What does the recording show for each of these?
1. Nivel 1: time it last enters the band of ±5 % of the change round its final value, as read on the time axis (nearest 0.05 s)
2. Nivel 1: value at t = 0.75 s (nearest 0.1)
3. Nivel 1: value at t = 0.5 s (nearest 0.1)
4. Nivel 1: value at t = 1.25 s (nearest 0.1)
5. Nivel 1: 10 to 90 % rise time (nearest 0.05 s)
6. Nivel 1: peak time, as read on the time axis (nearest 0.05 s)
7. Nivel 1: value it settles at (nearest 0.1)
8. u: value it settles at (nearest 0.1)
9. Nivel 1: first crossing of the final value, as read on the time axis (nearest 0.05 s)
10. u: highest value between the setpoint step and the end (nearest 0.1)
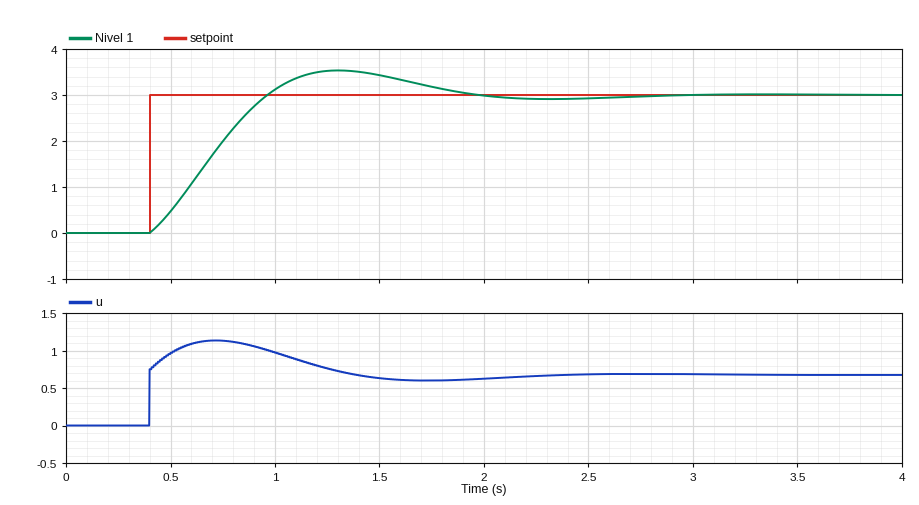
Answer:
1.80 s
2.0
0.5
3.5
0.40 s
1.30 s
3.0
0.7
0.95 s
1.1
